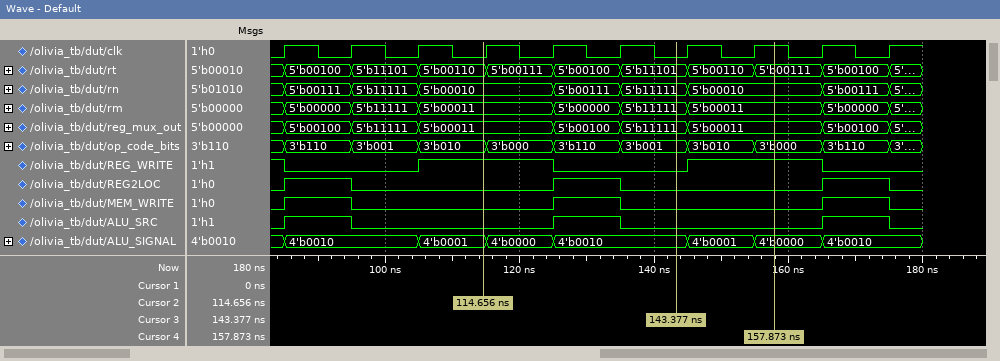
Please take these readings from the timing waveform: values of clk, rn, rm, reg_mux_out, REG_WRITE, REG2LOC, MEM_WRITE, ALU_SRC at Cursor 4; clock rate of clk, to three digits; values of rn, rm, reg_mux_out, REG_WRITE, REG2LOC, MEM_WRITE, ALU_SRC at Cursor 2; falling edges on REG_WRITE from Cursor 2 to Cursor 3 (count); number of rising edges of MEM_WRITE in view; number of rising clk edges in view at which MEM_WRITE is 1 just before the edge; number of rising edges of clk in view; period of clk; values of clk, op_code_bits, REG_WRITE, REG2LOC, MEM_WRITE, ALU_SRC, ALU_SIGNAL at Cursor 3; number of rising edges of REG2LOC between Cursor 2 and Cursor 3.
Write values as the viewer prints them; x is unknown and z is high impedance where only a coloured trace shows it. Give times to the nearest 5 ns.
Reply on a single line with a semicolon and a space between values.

clk=1, rn=5'b00010, rm=5'b00011, reg_mux_out=5'b00011, REG_WRITE=1, REG2LOC=0, MEM_WRITE=0, ALU_SRC=0; 100 MHz; rn=5'b00010, rm=5'b00011, reg_mux_out=5'b00011, REG_WRITE=1, REG2LOC=0, MEM_WRITE=0, ALU_SRC=0; 1; 3; 3; 10; 10 ns; clk=0, op_code_bits=3'b001, REG_WRITE=0, REG2LOC=0, MEM_WRITE=0, ALU_SRC=0, ALU_SIGNAL=4'b0010; 1
